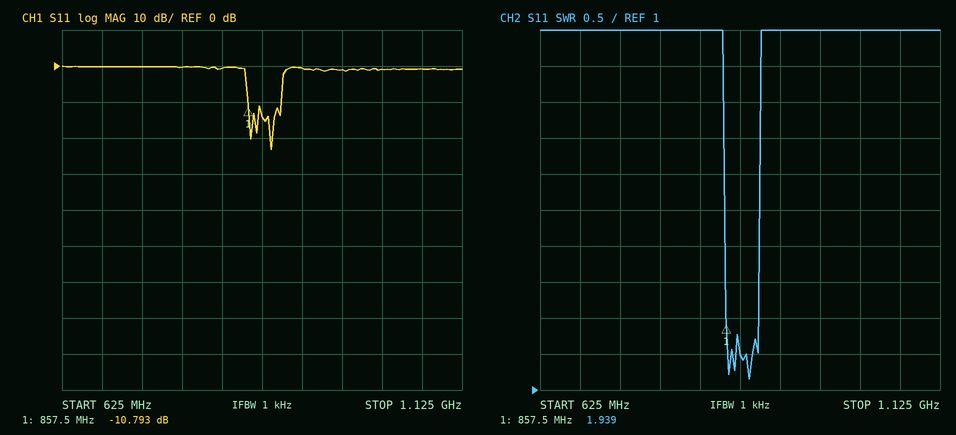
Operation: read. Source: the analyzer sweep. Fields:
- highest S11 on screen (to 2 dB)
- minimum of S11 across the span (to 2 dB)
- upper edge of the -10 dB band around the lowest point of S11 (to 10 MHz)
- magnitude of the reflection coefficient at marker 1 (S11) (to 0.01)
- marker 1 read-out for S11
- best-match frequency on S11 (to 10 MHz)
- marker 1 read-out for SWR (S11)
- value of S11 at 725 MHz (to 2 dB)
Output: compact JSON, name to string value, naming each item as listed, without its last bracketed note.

{"highest S11 on screen": "0 dB", "minimum of S11 across the span": "-24 dB", "upper edge of the -10 dB band around the lowest point of S11": "900 MHz", "magnitude of the reflection coefficient at marker 1 (S11)": "0.29", "marker 1 read-out for S11": "-10.793 dB", "best-match frequency on S11": "890 MHz", "marker 1 read-out for SWR": "1.939", "value of S11 at 725 MHz": "0 dB"}
